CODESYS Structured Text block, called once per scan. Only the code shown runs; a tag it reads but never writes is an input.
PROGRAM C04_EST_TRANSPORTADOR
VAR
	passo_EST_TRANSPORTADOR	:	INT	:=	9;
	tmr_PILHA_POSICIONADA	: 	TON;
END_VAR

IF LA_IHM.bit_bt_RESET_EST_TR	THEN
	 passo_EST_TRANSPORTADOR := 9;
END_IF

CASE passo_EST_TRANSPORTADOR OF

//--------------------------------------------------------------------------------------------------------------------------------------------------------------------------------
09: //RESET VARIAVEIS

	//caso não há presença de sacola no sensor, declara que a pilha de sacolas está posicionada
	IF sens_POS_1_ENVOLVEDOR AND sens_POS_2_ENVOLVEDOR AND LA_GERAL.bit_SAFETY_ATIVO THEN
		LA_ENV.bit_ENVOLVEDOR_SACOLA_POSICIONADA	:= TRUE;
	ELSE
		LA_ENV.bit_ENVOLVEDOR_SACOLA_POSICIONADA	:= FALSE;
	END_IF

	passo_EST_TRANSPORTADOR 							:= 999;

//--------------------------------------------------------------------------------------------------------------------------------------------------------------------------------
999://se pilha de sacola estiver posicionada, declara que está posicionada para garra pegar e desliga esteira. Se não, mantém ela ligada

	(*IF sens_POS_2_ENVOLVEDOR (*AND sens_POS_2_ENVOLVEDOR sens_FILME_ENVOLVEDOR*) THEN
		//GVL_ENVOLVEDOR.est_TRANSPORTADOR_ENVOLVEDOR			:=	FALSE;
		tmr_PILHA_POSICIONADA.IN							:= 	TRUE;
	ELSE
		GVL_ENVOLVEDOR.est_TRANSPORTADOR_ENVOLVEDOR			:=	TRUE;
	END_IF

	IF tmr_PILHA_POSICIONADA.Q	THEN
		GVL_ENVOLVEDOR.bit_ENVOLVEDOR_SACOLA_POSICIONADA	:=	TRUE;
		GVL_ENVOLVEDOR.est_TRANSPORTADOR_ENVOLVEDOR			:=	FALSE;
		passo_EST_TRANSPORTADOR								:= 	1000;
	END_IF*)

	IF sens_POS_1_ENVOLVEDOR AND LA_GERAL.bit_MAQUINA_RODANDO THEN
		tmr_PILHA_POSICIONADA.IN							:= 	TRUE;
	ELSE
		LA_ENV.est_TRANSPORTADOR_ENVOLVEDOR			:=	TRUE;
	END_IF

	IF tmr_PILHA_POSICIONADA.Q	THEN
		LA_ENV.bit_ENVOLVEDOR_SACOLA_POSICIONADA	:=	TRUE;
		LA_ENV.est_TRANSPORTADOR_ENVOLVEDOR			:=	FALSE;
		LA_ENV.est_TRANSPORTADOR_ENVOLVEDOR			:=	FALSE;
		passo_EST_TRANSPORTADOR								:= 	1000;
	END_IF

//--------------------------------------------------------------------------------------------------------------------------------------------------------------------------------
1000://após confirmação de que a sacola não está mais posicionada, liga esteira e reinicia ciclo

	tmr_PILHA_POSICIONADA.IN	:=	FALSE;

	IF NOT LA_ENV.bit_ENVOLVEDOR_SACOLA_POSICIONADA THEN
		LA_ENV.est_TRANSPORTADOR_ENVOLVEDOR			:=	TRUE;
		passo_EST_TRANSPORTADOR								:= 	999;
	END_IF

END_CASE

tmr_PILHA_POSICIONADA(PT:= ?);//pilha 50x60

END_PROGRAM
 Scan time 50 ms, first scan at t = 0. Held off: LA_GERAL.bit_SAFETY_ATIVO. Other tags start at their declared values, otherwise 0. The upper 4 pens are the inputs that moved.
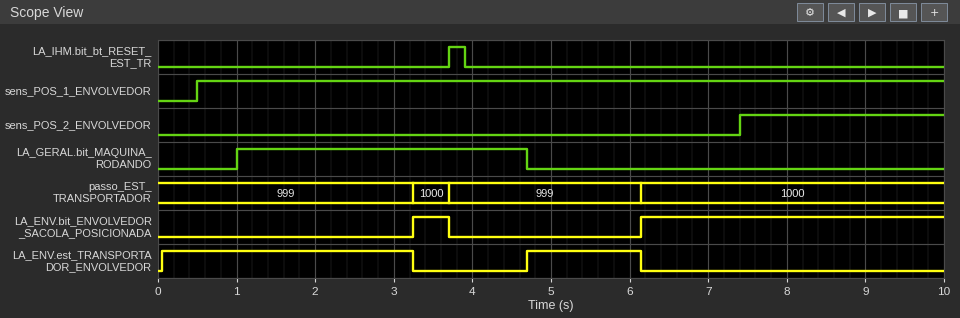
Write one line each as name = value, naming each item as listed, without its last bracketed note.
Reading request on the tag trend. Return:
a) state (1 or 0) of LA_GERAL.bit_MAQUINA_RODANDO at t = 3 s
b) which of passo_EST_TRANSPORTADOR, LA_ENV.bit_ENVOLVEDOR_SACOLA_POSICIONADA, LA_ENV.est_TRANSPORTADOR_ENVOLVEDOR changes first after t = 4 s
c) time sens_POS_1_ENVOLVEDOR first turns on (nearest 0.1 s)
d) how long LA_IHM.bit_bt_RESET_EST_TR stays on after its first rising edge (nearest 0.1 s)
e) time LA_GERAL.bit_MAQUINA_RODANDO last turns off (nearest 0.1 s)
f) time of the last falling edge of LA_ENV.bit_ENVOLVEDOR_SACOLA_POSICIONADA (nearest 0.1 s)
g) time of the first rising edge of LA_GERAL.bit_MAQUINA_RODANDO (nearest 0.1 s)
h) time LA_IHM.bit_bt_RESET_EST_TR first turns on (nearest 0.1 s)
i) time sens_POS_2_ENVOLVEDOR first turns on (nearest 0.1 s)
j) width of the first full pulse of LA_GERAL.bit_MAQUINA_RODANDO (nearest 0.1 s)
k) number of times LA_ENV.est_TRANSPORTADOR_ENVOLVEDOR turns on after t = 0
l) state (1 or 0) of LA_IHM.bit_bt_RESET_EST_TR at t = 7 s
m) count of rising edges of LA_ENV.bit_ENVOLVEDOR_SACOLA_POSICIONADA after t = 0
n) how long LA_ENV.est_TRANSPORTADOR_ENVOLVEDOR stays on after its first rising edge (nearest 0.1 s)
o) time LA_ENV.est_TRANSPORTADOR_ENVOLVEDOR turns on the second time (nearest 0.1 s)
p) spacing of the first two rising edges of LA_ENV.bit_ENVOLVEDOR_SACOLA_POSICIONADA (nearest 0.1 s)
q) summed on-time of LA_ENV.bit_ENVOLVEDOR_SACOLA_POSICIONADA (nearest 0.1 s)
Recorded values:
state (1 or 0) of LA_GERAL.bit_MAQUINA_RODANDO at t = 3 s = 1
which of passo_EST_TRANSPORTADOR, LA_ENV.bit_ENVOLVEDOR_SACOLA_POSICIONADA, LA_ENV.est_TRANSPORTADOR_ENVOLVEDOR changes first after t = 4 s = LA_ENV.est_TRANSPORTADOR_ENVOLVEDOR
time sens_POS_1_ENVOLVEDOR first turns on = 0.5 s
how long LA_IHM.bit_bt_RESET_EST_TR stays on after its first rising edge = 0.2 s
time LA_GERAL.bit_MAQUINA_RODANDO last turns off = 4.7 s
time of the last falling edge of LA_ENV.bit_ENVOLVEDOR_SACOLA_POSICIONADA = 3.7 s
time of the first rising edge of LA_GERAL.bit_MAQUINA_RODANDO = 1.0 s
time LA_IHM.bit_bt_RESET_EST_TR first turns on = 3.7 s
time sens_POS_2_ENVOLVEDOR first turns on = 7.4 s
width of the first full pulse of LA_GERAL.bit_MAQUINA_RODANDO = 3.7 s
number of times LA_ENV.est_TRANSPORTADOR_ENVOLVEDOR turns on after t = 0 = 2
state (1 or 0) of LA_IHM.bit_bt_RESET_EST_TR at t = 7 s = 0
count of rising edges of LA_ENV.bit_ENVOLVEDOR_SACOLA_POSICIONADA after t = 0 = 2
how long LA_ENV.est_TRANSPORTADOR_ENVOLVEDOR stays on after its first rising edge = 3.2 s
time LA_ENV.est_TRANSPORTADOR_ENVOLVEDOR turns on the second time = 4.7 s
spacing of the first two rising edges of LA_ENV.bit_ENVOLVEDOR_SACOLA_POSICIONADA = 2.9 s
summed on-time of LA_ENV.bit_ENVOLVEDOR_SACOLA_POSICIONADA = 4.3 s
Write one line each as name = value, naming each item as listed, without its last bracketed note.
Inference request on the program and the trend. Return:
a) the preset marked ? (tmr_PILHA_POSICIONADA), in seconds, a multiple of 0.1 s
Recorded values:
the preset marked ? (tmr_PILHA_POSICIONADA), in seconds, a multiple of 0.1 s = 2.2 s
